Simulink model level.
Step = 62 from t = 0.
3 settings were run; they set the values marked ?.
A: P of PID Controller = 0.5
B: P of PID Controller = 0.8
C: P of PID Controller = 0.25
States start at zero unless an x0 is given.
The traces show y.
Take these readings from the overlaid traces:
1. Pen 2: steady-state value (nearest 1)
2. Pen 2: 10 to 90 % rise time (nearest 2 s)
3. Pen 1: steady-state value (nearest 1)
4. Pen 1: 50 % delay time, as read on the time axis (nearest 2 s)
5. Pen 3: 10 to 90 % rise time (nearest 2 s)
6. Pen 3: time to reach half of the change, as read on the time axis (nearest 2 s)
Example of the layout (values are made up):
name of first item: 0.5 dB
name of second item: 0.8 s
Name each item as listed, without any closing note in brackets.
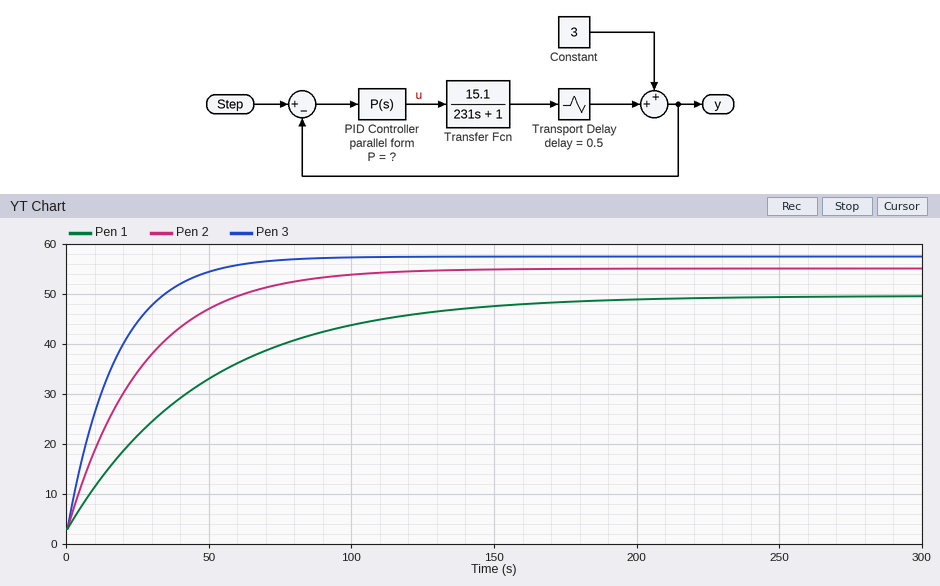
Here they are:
Pen 2: steady-state value: 55
Pen 2: 10 to 90 % rise time: 58 s
Pen 1: steady-state value: 50
Pen 1: 50 % delay time, as read on the time axis: 34 s
Pen 3: 10 to 90 % rise time: 38 s
Pen 3: time to reach half of the change, as read on the time axis: 12 s
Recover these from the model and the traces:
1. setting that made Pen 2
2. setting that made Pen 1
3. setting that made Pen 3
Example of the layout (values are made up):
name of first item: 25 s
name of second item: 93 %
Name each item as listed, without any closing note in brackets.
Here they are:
setting that made Pen 2: A
setting that made Pen 1: C
setting that made Pen 3: B
